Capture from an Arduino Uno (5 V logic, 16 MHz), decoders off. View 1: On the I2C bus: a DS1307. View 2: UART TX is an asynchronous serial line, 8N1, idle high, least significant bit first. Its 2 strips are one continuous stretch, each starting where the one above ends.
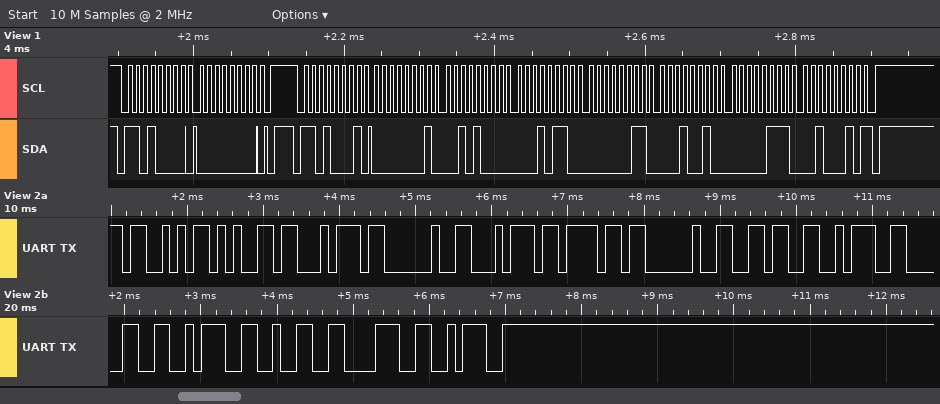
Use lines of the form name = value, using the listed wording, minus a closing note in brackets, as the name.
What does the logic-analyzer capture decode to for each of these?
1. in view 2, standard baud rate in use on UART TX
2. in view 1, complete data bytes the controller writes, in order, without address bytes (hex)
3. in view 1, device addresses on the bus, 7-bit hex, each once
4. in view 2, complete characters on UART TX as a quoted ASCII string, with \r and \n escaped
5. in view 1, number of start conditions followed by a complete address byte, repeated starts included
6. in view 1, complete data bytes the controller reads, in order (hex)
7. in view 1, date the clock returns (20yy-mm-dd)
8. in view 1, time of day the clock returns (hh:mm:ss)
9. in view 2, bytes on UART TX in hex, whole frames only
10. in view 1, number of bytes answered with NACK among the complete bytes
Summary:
in view 2, standard baud rate in use on UART TX = 9600 baud
in view 1, complete data bytes the controller writes, in order, without address bytes = 00
in view 1, device addresses on the bus, 7-bit hex, each once = 0x68
in view 2, complete characters on UART TX as a quoted ASCII string, with \r and \n escaped = "Set to 6:0:28:"
in view 1, number of start conditions followed by a complete address byte, repeated starts included = 2
in view 1, complete data bytes the controller reads, in order = 01 28 16 03 12 07 22
in view 1, date the clock returns = 2022-07-12
in view 1, time of day the clock returns = 16:28:01
in view 2, bytes on UART TX in hex, whole frames only = 0x53 0x65 0x74 0x20 0x74 0x6F 0x20 0x36 0x3A 0x30 0x3A 0x32 0x38 0x3A
in view 1, number of bytes answered with NACK among the complete bytes = 1
